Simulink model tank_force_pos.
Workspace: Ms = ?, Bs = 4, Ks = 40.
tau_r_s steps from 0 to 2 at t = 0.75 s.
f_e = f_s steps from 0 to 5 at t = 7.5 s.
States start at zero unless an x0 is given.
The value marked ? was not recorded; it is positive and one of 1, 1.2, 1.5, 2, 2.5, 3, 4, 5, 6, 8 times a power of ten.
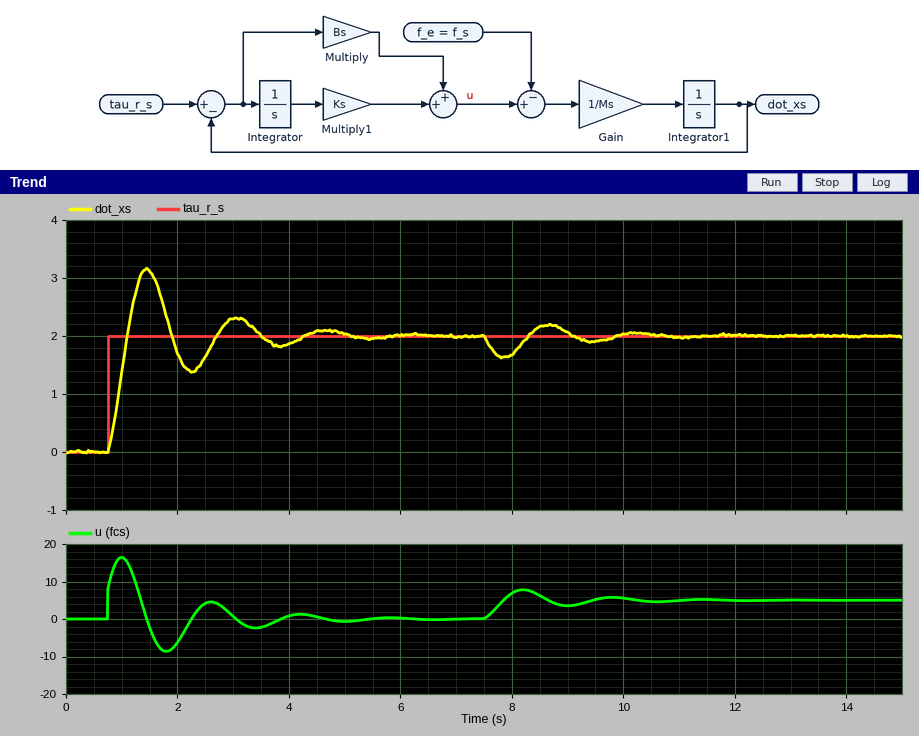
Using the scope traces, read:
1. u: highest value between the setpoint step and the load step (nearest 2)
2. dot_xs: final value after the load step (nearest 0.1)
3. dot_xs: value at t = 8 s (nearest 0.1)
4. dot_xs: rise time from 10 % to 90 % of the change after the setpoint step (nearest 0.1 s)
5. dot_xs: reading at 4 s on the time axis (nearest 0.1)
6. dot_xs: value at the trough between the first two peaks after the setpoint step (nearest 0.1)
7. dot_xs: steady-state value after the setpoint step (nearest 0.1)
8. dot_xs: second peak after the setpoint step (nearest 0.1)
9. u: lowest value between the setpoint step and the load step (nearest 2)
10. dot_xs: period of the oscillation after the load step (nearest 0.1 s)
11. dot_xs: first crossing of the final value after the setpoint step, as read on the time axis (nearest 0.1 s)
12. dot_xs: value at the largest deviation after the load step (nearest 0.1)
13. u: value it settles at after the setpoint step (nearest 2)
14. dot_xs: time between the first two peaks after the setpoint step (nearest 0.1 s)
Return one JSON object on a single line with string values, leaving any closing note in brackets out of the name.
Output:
{"u: highest value between the setpoint step and the load step": "16", "dot_xs: final value after the load step": "2.0", "dot_xs: value at t = 8 s": "1.7", "dot_xs: rise time from 10 % to 90 % of the change after the setpoint step": "0.3 s", "dot_xs: reading at 4 s on the time axis": "1.9", "dot_xs: value at the trough between the first two peaks after the setpoint step": "1.4", "dot_xs: steady-state value after the setpoint step": "2.0", "dot_xs: second peak after the setpoint step": "2.3", "u: lowest value between the setpoint step and the load step": "-8", "dot_xs: period of the oscillation after the load step": "1.6 s", "dot_xs: first crossing of the final value after the setpoint step, as read on the time axis": "1.1 s", "dot_xs: value at the largest deviation after the load step": "1.6", "u: value it settles at after the setpoint step": "0", "dot_xs: time between the first two peaks after the setpoint step": "1.6 s"}
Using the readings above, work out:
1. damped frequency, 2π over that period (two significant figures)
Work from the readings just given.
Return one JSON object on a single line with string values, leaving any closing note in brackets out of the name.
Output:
{"damped frequency, 2π over that period": "3.9 rad/s"}
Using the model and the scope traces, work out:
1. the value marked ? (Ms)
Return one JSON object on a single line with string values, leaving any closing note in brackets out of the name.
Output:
{"the value marked ?": "2.5"}
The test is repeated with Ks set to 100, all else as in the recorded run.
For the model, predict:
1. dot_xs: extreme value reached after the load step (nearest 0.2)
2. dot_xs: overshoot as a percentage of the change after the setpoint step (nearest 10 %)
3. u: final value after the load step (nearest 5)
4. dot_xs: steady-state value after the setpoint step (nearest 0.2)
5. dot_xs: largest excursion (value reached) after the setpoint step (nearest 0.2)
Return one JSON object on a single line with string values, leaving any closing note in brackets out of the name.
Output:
{"dot_xs: extreme value reached after the load step": "1.8", "dot_xs: overshoot as a percentage of the change after the setpoint step": "70 %", "u: final value after the load step": "5", "dot_xs: steady-state value after the setpoint step": "2.0", "dot_xs: largest excursion (value reached) after the setpoint step": "3.4"}
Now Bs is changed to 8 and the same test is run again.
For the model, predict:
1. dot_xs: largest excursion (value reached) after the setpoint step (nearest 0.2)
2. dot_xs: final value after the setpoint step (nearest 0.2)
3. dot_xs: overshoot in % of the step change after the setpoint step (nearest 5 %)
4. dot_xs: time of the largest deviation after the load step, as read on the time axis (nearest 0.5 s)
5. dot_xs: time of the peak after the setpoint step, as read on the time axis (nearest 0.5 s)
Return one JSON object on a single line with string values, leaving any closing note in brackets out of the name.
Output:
{"dot_xs: largest excursion (value reached) after the setpoint step": "2.8", "dot_xs: final value after the setpoint step": "2.0", "dot_xs: overshoot in % of the step change after the setpoint step": "35 %", "dot_xs: time of the largest deviation after the load step, as read on the time axis": "8.0 s", "dot_xs: time of the peak after the setpoint step, as read on the time axis": "1.5 s"}
